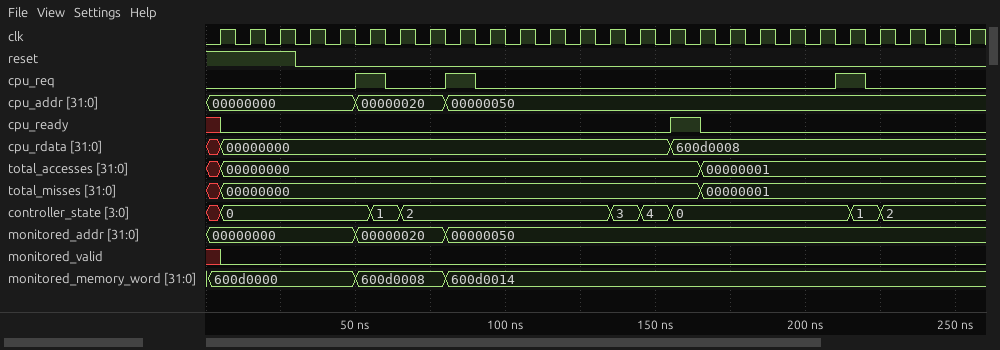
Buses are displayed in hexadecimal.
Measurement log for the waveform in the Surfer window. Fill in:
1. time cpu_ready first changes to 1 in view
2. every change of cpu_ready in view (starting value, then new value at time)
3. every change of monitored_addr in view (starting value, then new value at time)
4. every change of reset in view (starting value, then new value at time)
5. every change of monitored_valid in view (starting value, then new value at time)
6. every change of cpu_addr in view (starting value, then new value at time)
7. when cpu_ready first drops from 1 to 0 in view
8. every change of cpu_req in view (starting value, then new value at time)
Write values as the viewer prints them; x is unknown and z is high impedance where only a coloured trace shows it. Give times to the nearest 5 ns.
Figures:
155 ns
x, 0 at 5 ns, 1 at 155 ns, 0 at 165 ns
00000000, 00000020 at 50 ns, 00000050 at 80 ns
1, 0 at 30 ns
x, 0 at 5 ns
00000000, 00000020 at 50 ns, 00000050 at 80 ns
165 ns
0, 1 at 50 ns, 0 at 60 ns, 1 at 80 ns, 0 at 90 ns, 1 at 210 ns, 0 at 220 ns
